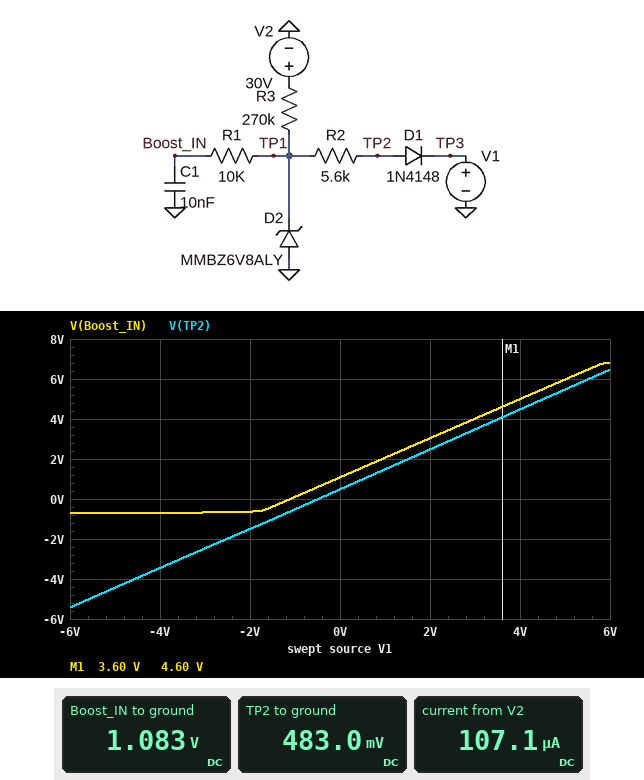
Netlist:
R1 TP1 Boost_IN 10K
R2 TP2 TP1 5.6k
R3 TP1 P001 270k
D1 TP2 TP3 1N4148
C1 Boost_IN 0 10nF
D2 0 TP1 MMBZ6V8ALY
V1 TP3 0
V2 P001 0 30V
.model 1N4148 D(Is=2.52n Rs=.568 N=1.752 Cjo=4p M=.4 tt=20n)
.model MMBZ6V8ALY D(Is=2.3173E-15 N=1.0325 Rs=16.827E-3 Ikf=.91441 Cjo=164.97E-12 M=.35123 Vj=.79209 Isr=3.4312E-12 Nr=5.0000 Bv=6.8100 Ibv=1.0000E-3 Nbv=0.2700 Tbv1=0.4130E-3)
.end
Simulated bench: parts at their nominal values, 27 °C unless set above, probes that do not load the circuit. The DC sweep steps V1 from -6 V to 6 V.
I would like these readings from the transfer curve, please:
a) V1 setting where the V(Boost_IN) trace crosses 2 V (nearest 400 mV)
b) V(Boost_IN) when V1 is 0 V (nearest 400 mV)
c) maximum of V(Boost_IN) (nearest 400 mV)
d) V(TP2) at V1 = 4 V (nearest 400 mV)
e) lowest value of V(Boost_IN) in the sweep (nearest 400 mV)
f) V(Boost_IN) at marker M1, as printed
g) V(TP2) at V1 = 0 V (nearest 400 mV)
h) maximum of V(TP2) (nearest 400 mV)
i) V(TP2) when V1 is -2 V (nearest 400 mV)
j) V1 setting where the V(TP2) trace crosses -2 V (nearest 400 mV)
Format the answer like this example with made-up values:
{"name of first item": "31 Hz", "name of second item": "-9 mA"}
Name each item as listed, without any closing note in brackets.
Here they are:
{"V1 setting where the V(Boost_IN) trace crosses 2 V": "800 mV", "V(Boost_IN) when V1 is 0 V": "1.2 V", "maximum of V(Boost_IN)": "6.8 V", "V(TP2) at V1 = 4 V": "4.4 V", "lowest value of V(Boost_IN) in the sweep": "-800 mV", "V(Boost_IN) at marker M1, as printed": "4.60 V", "V(TP2) at V1 = 0 V": "400 mV", "maximum of V(TP2)": "6.4 V", "V(TP2) when V1 is -2 V": "-1.6 V", "V1 setting where the V(TP2) trace crosses -2 V": "-2.4 V"}
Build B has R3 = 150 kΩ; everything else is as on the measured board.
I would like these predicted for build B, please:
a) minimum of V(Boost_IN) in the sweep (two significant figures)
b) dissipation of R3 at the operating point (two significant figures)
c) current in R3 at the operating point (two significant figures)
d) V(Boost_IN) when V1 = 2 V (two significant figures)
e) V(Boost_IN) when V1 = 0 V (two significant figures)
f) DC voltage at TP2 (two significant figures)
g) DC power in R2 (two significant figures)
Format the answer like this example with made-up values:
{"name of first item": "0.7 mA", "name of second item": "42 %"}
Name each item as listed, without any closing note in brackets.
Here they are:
{"minimum of V(Boost_IN) in the sweep": "-700 mV", "dissipation of R3 at the operating point": "5.4 mW", "current in R3 at the operating point": "190 µA", "V(Boost_IN) when V1 = 2 V": "3.5 V", "V(Boost_IN) when V1 = 0 V": "1.6 V", "DC voltage at TP2": "510 mV", "DC power in R2": "200 µW"}
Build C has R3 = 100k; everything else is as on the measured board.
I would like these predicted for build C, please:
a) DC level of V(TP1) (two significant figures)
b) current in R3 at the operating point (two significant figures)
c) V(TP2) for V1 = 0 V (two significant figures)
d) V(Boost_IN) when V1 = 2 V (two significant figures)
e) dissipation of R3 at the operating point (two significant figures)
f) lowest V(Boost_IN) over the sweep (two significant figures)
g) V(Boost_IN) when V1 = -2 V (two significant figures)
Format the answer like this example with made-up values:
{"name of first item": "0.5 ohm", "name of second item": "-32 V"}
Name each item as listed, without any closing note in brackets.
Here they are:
{"DC level of V(TP1)": "2.1 V", "current in R3 at the operating point": "280 µA", "V(TP2) for V1 = 0 V": "530 mV", "V(Boost_IN) when V1 = 2 V": "4.0 V", "dissipation of R3 at the operating point": "7.8 mW", "lowest V(Boost_IN) over the sweep": "-700 mV", "V(Boost_IN) when V1 = -2 V": "200 mV"}
